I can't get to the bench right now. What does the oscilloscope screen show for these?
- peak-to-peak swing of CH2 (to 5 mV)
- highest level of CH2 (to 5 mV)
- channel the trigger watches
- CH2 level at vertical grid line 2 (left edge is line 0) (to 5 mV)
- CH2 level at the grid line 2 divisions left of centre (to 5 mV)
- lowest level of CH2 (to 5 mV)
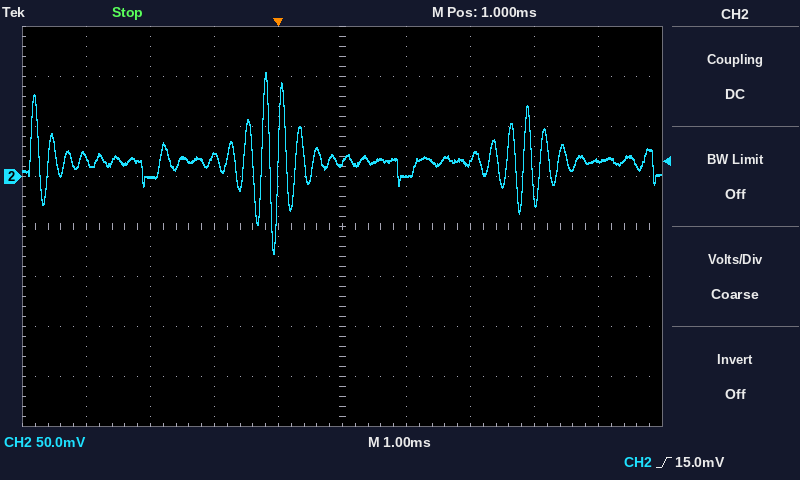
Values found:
180 mV
105 mV
CH2
0 mV
20 mV
-75 mV
